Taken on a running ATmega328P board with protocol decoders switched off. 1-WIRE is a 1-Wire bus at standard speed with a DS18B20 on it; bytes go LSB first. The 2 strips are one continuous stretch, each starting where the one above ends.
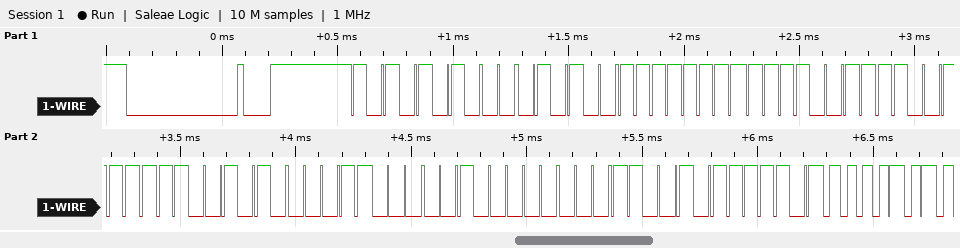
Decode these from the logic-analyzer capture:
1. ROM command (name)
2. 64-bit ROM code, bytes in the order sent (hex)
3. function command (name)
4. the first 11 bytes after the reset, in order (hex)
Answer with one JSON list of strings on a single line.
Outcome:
["Match ROM", "28 FF CF F3 53 18 04 98", "Read Scratchpad", "55 28 FF CF F3 53 18 04 98 BE 50"]
